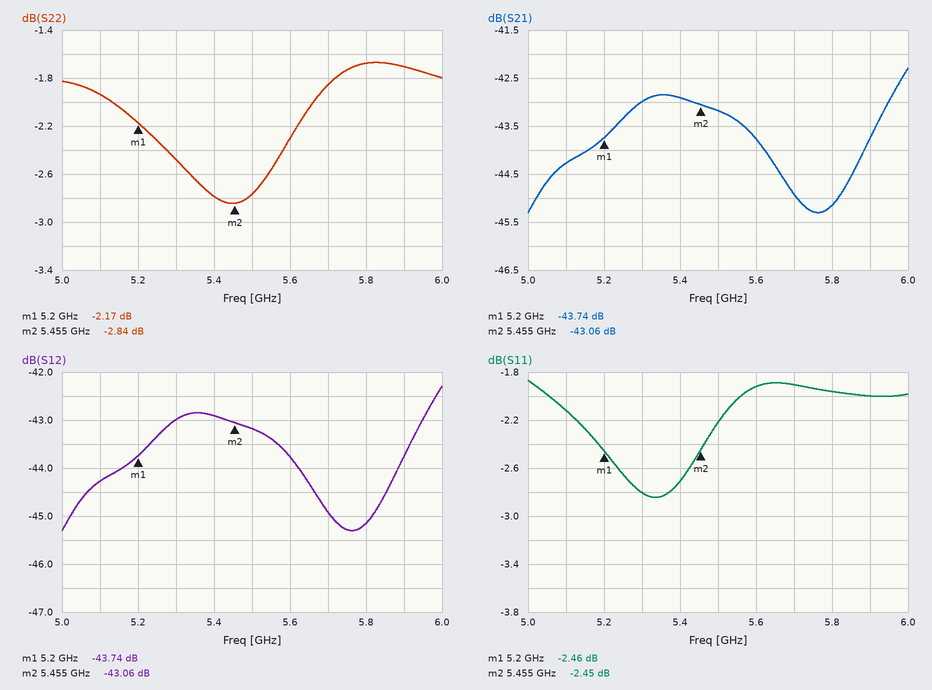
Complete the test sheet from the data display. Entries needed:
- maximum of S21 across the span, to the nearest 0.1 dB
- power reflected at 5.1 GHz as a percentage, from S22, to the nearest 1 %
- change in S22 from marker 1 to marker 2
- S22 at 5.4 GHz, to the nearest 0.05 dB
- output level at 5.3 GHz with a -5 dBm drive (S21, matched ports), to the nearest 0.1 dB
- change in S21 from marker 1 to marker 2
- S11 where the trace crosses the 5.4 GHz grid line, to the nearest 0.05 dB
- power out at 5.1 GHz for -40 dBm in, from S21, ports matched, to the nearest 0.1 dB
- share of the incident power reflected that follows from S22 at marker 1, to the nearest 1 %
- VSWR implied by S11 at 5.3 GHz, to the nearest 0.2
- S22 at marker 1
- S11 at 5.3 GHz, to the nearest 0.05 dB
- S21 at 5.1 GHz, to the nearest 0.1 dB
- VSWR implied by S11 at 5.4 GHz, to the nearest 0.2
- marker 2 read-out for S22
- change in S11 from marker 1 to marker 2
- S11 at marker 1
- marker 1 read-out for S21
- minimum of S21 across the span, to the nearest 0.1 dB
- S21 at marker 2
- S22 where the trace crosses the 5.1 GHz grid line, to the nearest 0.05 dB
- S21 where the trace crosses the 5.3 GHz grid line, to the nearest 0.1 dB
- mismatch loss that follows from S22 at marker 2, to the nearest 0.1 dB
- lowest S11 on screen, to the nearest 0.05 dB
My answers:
-42.3 dB
64 %
-0.67 dB
-2.80 dB
-48.0 dBm
0.68 dB
-2.70 dB
-84.3 dBm
61 %
6.2
-2.17 dB
-2.80 dB
-44.3 dB
6.4
-2.84 dB
0.01 dB
-2.46 dB
-43.74 dB
-45.3 dB
-43.06 dB
-1.95 dB
-43.0 dB
3.2 dB
-2.85 dB
